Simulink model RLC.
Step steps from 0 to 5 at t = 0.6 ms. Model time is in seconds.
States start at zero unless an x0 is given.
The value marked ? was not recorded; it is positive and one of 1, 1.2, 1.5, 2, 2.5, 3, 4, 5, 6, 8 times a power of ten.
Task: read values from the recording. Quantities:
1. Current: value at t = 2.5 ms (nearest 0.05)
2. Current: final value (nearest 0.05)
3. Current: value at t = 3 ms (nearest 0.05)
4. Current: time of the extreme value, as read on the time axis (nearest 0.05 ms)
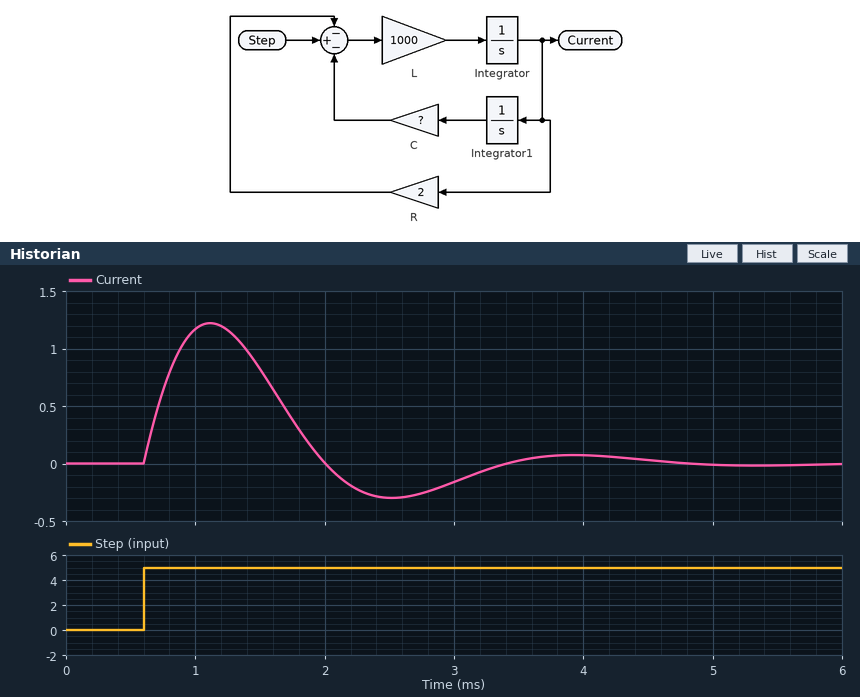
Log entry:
-0.30
0.00
-0.15
1.10 ms
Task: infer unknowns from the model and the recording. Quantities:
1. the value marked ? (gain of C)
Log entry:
6000
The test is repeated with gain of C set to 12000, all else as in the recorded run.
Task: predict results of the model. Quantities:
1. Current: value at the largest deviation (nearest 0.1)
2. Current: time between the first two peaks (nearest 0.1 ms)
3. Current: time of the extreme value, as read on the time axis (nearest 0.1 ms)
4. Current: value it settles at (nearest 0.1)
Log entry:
1.0
1.9 ms
1.0 ms
0.0
